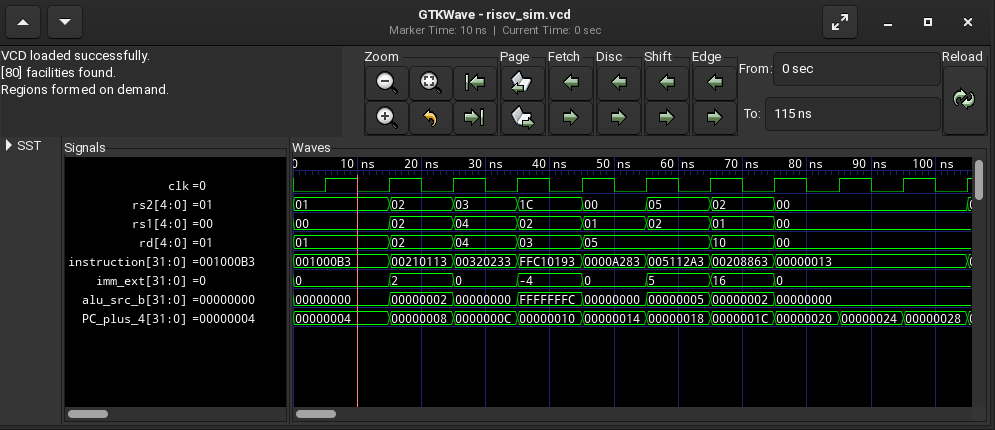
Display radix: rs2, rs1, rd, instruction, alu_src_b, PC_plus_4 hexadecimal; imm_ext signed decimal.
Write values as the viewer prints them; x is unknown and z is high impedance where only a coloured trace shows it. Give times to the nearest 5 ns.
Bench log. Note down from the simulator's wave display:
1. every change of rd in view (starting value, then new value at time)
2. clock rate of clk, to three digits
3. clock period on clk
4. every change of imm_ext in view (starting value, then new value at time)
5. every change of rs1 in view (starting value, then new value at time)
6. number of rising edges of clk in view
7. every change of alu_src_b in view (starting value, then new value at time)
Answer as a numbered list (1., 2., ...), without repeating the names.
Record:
1. 01, 02 at 15 ns, 04 at 25 ns, 03 at 35 ns, 05 at 45 ns, 10 at 65 ns, 00 at 75 ns
2. 100 MHz
3. 10 ns
4. 0, 2 at 15 ns, 0 at 25 ns, -4 at 35 ns, 0 at 45 ns, 5 at 55 ns, 16 at 65 ns, 0 at 75 ns
5. 00, 02 at 15 ns, 04 at 25 ns, 02 at 35 ns, 01 at 45 ns, 02 at 55 ns, 01 at 65 ns, 00 at 75 ns
6. 11
7. 00000000, 00000002 at 15 ns, 00000000 at 25 ns, FFFFFFFC at 35 ns, 00000000 at 45 ns, 00000005 at 55 ns, 00000002 at 65 ns, 00000000 at 75 ns
